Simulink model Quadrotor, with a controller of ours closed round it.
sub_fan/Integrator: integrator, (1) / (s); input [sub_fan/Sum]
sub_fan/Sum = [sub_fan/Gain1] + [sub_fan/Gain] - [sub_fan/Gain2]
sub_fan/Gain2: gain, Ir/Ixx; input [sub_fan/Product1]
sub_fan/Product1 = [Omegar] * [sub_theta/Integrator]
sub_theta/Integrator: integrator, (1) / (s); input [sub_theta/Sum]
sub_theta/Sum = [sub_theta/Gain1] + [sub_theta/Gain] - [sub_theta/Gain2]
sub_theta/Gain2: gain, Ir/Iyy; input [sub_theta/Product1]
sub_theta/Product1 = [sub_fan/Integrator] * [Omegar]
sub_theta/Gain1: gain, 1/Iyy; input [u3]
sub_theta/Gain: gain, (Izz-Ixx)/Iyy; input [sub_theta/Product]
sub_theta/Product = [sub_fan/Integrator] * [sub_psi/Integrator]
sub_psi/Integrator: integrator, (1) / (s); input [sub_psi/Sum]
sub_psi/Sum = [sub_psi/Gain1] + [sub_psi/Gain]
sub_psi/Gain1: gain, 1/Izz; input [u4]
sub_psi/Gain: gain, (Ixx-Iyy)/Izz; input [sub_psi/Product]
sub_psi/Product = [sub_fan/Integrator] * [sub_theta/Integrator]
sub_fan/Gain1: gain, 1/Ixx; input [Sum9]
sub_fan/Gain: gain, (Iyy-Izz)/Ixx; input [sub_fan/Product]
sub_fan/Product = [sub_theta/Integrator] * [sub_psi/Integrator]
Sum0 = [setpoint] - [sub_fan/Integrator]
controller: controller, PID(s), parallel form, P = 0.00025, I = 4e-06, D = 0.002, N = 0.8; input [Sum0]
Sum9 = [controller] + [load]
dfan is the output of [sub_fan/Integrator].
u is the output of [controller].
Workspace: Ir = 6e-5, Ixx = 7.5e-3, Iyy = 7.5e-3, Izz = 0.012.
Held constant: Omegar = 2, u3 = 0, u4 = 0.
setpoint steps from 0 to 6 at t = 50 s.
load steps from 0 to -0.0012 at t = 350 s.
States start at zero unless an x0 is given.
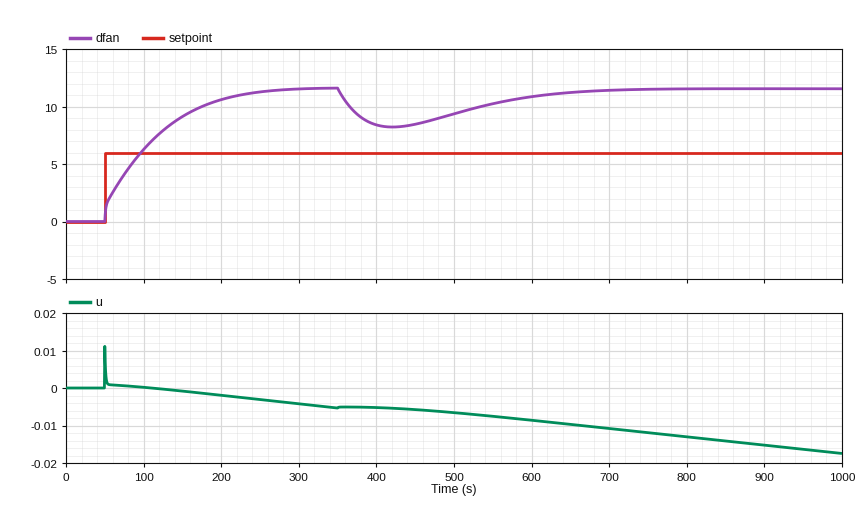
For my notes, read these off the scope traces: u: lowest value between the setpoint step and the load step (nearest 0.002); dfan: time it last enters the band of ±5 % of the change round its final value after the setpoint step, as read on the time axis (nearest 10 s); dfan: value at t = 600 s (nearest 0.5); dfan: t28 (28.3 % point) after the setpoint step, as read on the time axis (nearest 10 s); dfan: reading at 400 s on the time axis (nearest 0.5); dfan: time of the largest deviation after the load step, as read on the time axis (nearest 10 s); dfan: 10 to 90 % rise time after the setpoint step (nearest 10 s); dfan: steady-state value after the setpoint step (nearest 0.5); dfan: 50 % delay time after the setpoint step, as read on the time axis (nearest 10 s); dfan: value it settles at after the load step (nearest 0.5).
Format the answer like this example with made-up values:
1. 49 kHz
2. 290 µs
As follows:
1. -0.006
2. 220 s
3. 11.0
4. 70 s
5. 8.5
6. 420 s
7. 140 s
8. 11.5
9. 90 s
10. 11.5
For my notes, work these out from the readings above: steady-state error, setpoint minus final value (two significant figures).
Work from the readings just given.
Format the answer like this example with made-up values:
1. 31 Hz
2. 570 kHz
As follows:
1. -5.5
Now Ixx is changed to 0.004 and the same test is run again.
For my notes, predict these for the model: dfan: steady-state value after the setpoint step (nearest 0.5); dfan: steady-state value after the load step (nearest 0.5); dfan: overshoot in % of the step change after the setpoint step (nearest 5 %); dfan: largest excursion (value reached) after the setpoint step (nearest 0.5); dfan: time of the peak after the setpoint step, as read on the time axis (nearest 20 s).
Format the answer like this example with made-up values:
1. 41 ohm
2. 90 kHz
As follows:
1. 6.0
2. 6.0
3. 10 %
4. 6.5
5. 140 s
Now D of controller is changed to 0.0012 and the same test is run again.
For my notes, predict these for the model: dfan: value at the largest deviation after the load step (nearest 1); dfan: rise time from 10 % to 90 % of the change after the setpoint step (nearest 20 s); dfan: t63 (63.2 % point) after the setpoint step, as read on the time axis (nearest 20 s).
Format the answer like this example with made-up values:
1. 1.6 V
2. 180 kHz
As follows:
1. 8
2. 140 s
3. 120 s
